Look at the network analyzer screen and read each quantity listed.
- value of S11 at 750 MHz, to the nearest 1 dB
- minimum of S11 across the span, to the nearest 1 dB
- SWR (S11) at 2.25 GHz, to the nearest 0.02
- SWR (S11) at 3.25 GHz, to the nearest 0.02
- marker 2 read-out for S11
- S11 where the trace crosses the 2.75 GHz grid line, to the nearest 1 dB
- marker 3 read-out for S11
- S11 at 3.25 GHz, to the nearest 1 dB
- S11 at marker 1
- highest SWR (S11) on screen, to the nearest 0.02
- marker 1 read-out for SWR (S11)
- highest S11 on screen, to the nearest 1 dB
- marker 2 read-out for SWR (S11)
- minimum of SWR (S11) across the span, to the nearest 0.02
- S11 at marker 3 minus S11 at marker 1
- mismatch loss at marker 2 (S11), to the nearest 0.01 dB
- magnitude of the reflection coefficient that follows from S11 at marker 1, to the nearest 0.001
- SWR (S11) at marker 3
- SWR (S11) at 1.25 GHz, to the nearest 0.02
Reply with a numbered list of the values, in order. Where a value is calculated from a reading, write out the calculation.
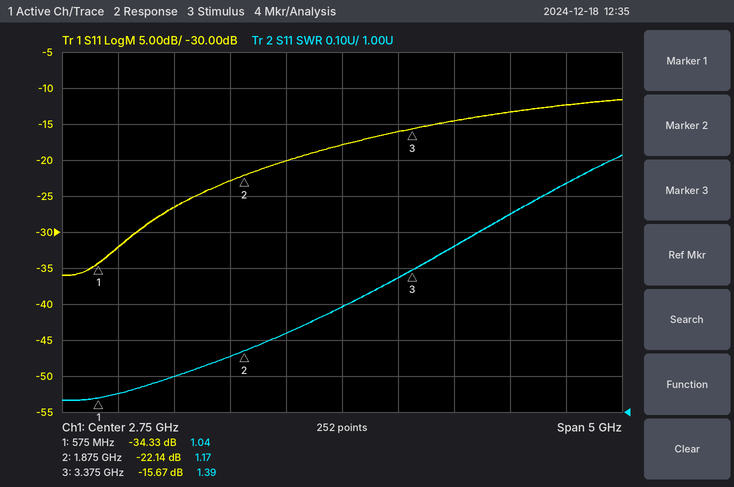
1. -32 dB
2. -36 dB
3. 1.22
4. 1.38
5. -22.14 dB
6. -18 dB
7. -15.67 dB
8. -16 dB
9. -34.33 dB
10. 1.72
11. 1.04
12. -12 dB
13. 1.17
14. 1.04
15. -15.67 − (-34.33) = 18.66 dB
16. −10 log10(1 − 10^(-22.14/10)) ≈ 0.03 dB
17. 10^(-34.33/20) ≈ 0.019
18. 1.39
19. 1.10
